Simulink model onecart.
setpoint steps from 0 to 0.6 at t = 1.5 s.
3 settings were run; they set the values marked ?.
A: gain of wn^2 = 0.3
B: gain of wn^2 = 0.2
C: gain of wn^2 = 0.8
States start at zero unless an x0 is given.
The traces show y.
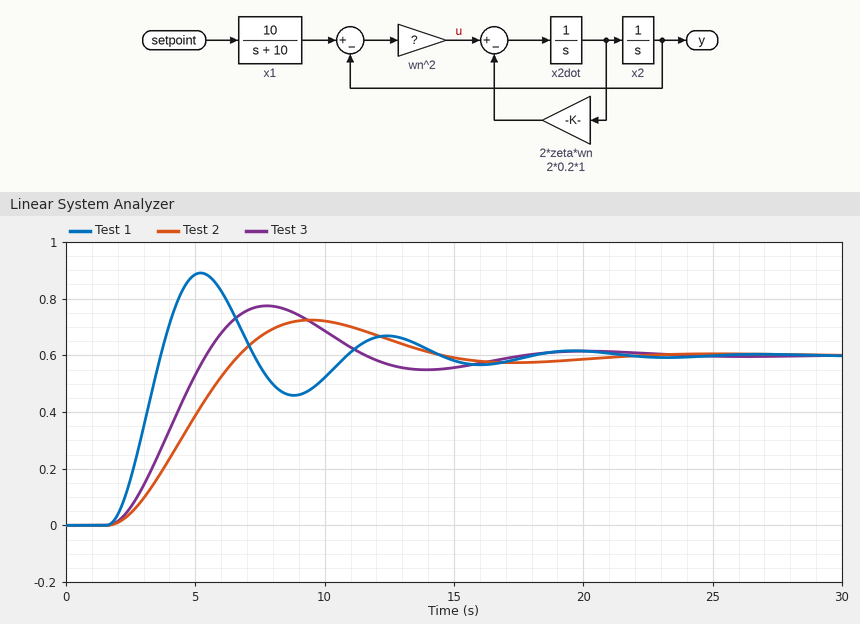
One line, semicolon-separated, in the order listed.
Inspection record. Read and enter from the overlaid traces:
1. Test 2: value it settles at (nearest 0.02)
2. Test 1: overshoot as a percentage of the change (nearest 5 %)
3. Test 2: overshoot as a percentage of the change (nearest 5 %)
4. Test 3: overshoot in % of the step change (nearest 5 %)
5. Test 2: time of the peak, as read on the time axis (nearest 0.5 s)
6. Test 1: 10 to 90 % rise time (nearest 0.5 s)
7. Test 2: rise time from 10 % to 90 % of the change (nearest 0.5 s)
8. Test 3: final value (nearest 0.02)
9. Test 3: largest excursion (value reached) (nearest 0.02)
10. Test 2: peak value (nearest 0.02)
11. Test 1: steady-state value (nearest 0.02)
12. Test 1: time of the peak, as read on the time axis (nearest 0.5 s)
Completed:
0.60; 50 %; 20 %; 30 %; 9.5 s; 1.5 s; 3.5 s; 0.60; 0.78; 0.72; 0.60; 5.0 s
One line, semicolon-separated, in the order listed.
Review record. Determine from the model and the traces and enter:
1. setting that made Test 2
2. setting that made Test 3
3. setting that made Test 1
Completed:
B; A; C
